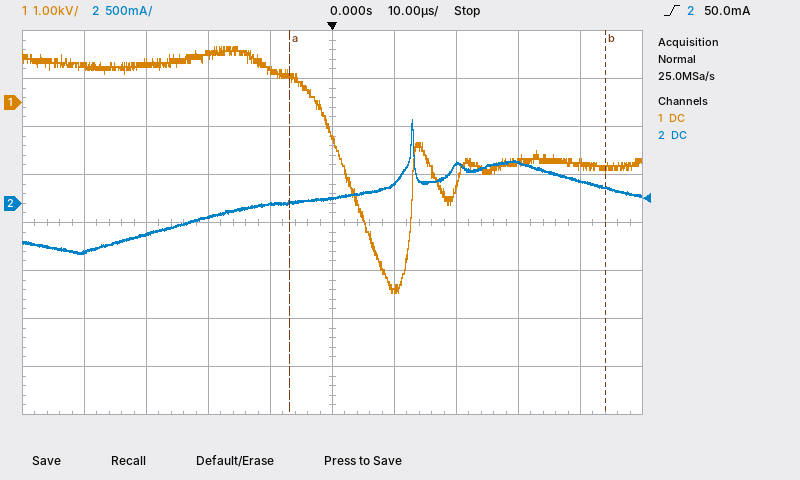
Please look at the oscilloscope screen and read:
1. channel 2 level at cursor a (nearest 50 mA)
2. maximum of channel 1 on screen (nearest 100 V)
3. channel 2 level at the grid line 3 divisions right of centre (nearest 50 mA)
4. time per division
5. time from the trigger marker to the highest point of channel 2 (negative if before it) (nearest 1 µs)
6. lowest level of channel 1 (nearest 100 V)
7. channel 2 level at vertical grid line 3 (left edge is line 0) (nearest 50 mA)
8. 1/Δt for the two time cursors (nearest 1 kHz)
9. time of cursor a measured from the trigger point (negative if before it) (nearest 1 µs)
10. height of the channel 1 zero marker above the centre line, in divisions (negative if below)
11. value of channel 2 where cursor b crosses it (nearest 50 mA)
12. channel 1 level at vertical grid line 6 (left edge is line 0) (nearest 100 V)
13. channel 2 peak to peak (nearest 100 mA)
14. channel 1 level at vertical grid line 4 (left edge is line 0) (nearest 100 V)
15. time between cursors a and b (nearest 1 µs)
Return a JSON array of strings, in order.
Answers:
["0 mA", "1.2 kV", "450 mA", "10 µs", "+13 µs", "-4.0 kV", "-150 mA", "20 kHz", "-7 µs", "+2.5 div", "150 mA", "-3.9 kV", "1.40 A", "700 V", "51 µs"]
